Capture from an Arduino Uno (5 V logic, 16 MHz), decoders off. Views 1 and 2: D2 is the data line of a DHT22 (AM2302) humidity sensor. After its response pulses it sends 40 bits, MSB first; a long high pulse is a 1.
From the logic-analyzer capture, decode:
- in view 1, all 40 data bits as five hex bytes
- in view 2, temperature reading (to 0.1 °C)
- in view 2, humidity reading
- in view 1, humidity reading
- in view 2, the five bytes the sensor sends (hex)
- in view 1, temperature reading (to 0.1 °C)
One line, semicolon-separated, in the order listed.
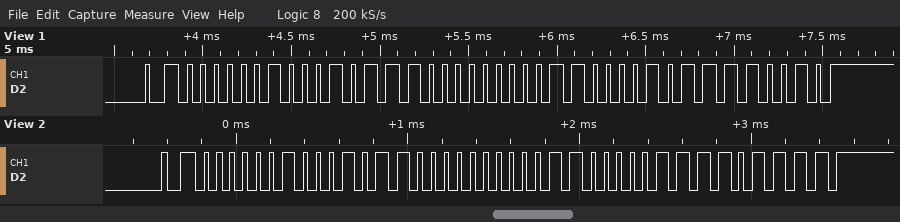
02 2E 00 C2 F2; 19.3 °C; 55.6 %; 55.8 %; 02 2C 00 C1 EF; 19.4 °C
